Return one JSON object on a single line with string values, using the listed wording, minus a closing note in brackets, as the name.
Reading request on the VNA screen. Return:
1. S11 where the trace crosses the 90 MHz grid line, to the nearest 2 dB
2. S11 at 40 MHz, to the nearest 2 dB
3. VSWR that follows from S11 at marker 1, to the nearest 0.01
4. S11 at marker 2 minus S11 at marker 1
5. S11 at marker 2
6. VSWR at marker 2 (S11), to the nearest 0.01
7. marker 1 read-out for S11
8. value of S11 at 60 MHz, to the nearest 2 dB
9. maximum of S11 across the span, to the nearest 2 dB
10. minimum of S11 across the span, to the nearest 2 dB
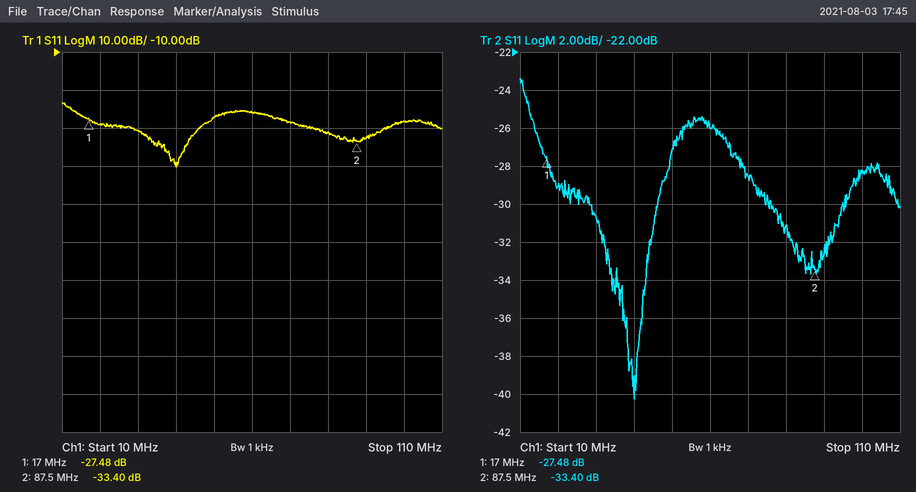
{"S11 where the trace crosses the 90 MHz grid line, to the nearest 2 dB": "-32 dB", "S11 at 40 MHz, to the nearest 2 dB": "-40 dB", "VSWR that follows from S11 at marker 1, to the nearest 0.01": "1.09", "S11 at marker 2 minus S11 at marker 1": "-5.92 dB", "S11 at marker 2": "-33.40 dB", "VSWR at marker 2 (S11), to the nearest 0.01": "1.04", "marker 1 read-out for S11": "-27.48 dB", "value of S11 at 60 MHz, to the nearest 2 dB": "-26 dB", "maximum of S11 across the span, to the nearest 2 dB": "-24 dB", "minimum of S11 across the span, to the nearest 2 dB": "-40 dB"}
